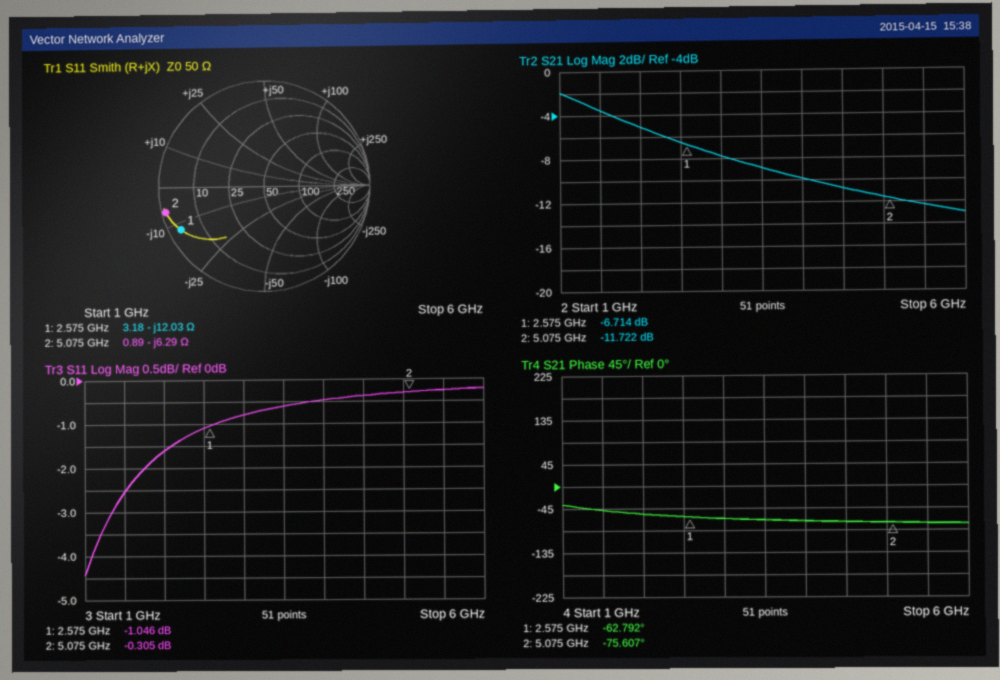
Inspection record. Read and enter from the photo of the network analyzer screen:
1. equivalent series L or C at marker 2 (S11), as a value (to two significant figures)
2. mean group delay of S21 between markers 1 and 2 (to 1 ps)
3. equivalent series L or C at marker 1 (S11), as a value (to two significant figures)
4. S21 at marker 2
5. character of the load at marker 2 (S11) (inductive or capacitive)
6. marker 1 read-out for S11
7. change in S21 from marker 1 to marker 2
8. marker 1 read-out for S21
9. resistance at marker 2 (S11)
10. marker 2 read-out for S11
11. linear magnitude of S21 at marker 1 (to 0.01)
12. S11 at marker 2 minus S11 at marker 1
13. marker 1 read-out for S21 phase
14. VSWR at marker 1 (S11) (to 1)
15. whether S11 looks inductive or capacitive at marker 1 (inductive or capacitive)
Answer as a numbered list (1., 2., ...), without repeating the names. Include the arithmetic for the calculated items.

1. C = 1/(2π × 5.075 GHz × 6.29 Ω) ≈ 5.0 pF
2. −(-75.607° − (-62.792°))/(360° × 2.5 GHz) ≈ 14 ps
3. C = 1/(2π × 2.575 GHz × 12.03 Ω) ≈ 5.1 pF
4. -11.722 dB
5. capacitive
6. -1.046 dB
7. -11.722 − (-6.714) = -5.008 dB
8. -6.714 dB
9. 0.89 Ω
10. -0.305 dB
11. 10^(-6.714/20) ≈ 0.46
12. -0.305 − (-1.046) = 0.741 dB
13. -62.792°
14. (1 + 0.8865)/(1 − 0.8865) ≈ 17
15. capacitive
